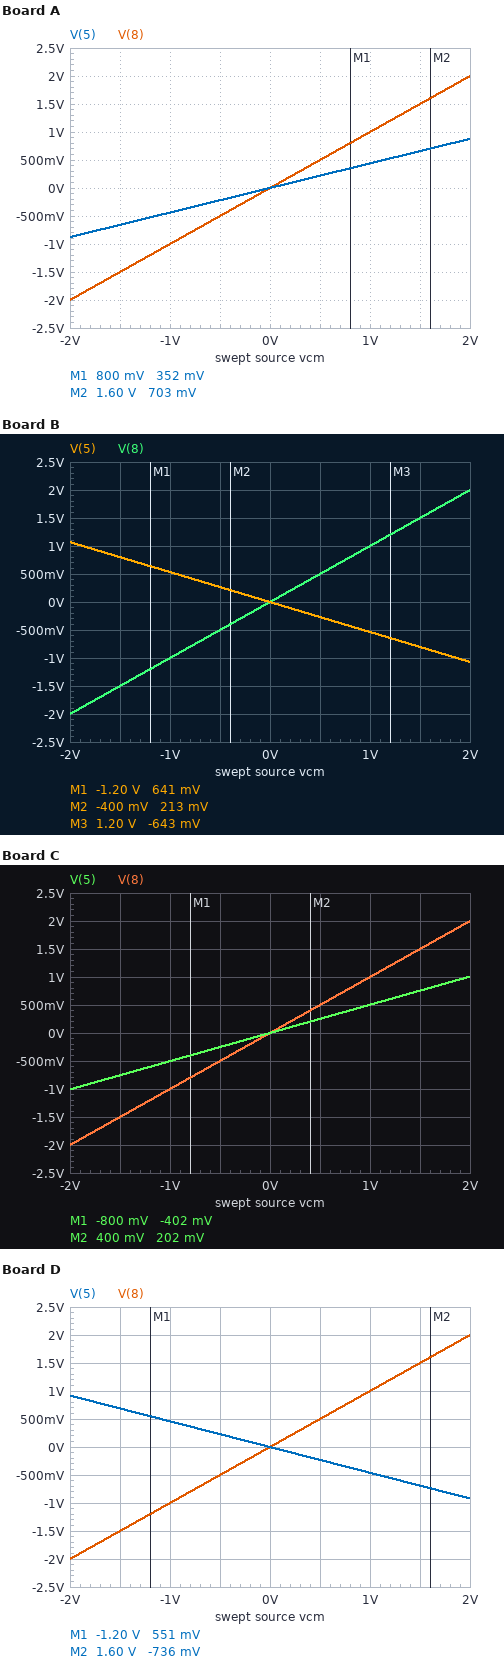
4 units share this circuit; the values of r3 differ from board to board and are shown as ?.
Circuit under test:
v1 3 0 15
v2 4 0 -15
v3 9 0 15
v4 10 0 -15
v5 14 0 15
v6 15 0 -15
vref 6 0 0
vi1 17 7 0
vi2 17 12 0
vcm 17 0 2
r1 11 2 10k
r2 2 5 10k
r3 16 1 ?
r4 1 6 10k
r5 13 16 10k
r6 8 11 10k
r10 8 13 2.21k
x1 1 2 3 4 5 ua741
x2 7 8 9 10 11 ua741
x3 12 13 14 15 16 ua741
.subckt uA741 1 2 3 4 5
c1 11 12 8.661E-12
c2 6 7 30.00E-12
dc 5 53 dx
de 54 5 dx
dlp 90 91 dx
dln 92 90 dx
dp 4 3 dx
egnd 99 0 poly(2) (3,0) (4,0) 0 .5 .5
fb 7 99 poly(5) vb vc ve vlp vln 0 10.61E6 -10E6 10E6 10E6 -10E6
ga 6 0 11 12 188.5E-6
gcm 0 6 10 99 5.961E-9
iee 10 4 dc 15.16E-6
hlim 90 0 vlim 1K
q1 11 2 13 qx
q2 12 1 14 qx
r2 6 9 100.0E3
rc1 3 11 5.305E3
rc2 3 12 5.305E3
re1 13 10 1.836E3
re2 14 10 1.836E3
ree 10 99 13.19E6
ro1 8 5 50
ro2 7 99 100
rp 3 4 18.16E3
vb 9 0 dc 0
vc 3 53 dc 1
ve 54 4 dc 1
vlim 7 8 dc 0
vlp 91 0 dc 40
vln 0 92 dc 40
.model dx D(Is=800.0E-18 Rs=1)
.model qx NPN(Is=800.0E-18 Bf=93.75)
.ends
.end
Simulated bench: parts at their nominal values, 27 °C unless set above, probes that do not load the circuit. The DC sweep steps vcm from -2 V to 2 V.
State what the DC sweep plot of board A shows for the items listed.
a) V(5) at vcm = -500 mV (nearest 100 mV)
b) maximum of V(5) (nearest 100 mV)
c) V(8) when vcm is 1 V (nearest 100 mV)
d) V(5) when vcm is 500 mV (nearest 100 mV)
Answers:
-200 mV
900 mV
1.0 V
200 mV
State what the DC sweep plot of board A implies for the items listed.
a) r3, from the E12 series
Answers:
3.9 kΩ
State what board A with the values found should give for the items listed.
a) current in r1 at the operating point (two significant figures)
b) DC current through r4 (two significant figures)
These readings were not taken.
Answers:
56 µA
140 µA
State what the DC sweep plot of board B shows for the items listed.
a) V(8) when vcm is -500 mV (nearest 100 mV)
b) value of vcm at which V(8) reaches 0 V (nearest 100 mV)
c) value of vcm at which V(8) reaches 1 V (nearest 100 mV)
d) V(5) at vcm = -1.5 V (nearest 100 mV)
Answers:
-500 mV
0 V
1.0 V
800 mV
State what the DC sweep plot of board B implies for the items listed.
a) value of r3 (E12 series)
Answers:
33 kΩ
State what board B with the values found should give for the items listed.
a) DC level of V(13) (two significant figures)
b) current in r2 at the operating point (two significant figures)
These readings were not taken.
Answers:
2.0 V
150 µA
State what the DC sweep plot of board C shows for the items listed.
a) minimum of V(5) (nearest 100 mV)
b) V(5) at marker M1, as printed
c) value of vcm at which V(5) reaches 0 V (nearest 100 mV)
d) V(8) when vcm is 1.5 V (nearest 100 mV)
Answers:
-1.0 V
-402 mV
0 V
1.5 V
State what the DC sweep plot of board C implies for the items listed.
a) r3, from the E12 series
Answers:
3.3 kΩ
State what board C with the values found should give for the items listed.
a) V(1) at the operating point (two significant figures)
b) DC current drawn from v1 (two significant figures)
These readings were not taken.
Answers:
1.5 V
1.7 mA
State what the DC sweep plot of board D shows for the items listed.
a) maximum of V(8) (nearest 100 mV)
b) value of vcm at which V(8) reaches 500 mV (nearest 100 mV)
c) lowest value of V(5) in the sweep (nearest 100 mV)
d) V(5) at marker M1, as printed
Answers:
2.0 V
500 mV
-900 mV
551 mV
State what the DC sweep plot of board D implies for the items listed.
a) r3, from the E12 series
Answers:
27 kΩ
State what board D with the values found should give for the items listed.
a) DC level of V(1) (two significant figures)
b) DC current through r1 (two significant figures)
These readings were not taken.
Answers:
540 mV
150 µA
